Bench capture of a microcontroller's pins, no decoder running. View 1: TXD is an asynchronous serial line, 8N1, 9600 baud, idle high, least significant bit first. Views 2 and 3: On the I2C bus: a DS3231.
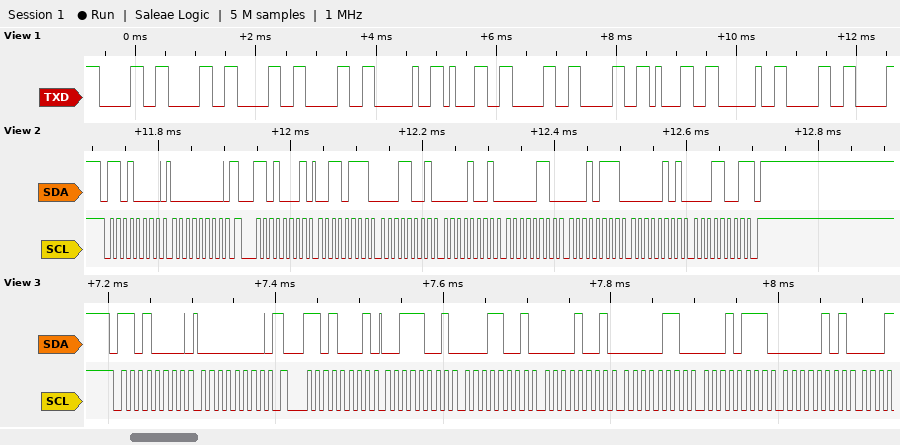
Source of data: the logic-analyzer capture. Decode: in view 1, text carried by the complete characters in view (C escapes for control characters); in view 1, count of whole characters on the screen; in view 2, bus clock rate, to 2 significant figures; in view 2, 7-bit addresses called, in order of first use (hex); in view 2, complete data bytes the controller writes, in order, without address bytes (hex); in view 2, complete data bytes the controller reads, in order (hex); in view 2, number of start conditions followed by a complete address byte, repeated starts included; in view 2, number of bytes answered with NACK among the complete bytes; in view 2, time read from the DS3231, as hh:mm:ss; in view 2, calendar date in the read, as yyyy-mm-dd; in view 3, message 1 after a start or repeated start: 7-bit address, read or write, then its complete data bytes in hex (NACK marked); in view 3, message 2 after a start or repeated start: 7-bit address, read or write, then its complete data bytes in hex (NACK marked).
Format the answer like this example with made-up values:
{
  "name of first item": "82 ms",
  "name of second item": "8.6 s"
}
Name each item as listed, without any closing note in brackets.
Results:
{
  "in view 1, text carried by the complete characters in view": "\"0000 1001 0\"",
  "in view 1, count of whole characters on the screen": "11",
  "in view 2, bus clock rate, to 2 significant figures": "100 kHz",
  "in view 2, 7-bit addresses called, in order of first use": "0x68",
  "in view 2, complete data bytes the controller writes, in order, without address bytes": "00",
  "in view 2, complete data bytes the controller reads, in order": "37 19 09 06 17 05 19",
  "in view 2, number of start conditions followed by a complete address byte, repeated starts included": "2",
  "in view 2, number of bytes answered with NACK among the complete bytes": "1",
  "in view 2, time read from the DS3231, as hh:mm:ss": "09:19:37",
  "in view 2, calendar date in the read, as yyyy-mm-dd": "2019-05-17",
  "in view 3, message 1 after a start or repeated start: 7-bit address, read or write, then its complete data bytes in hex": "0x68 write: 00",
  "in view 3, message 2 after a start or repeated start: 7-bit address, read or write, then its complete data bytes in hex": "0x68 read: 39 19 09 06 17 05"
}
